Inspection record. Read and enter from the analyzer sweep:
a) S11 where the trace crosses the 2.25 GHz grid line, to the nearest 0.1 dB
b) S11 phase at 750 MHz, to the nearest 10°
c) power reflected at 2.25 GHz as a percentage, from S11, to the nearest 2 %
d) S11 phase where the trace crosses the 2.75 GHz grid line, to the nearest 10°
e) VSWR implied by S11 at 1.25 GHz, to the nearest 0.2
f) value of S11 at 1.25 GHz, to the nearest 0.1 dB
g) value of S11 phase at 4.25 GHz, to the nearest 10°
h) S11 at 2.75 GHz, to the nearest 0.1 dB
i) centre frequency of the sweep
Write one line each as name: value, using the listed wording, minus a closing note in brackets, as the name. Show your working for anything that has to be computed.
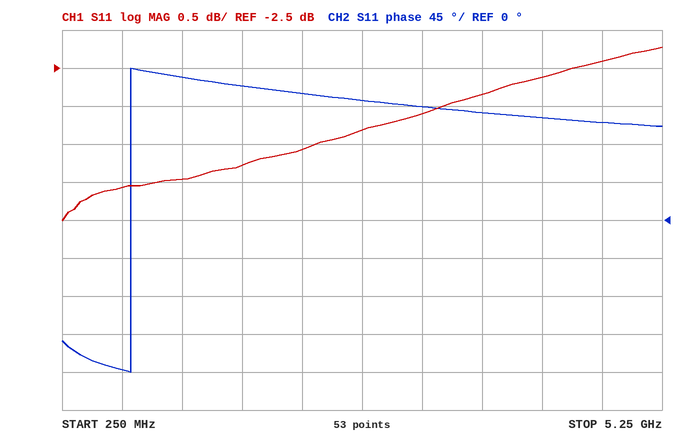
S11 where the trace crosses the 2.25 GHz grid line, to the nearest 0.1 dB: -3.6 dB
S11 phase at 750 MHz, to the nearest 10°: -180°
power reflected at 2.25 GHz as a percentage, from S11, to the nearest 2 %: 10^(-3.6/10) ≈ 44 %
S11 phase where the trace crosses the 2.75 GHz grid line, to the nearest 10°: 140°
VSWR implied by S11 at 1.25 GHz, to the nearest 0.2: |Γ| = 10^(-4/20) = 0.6310; VSWR = (1 + 0.6310)/(1 − 0.6310) ≈ 4.4
value of S11 at 1.25 GHz, to the nearest 0.1 dB: -4.0 dB
value of S11 phase at 4.25 GHz, to the nearest 10°: 120°
S11 at 2.75 GHz, to the nearest 0.1 dB: -3.3 dB
centre frequency of the sweep: 2.75 GHz
